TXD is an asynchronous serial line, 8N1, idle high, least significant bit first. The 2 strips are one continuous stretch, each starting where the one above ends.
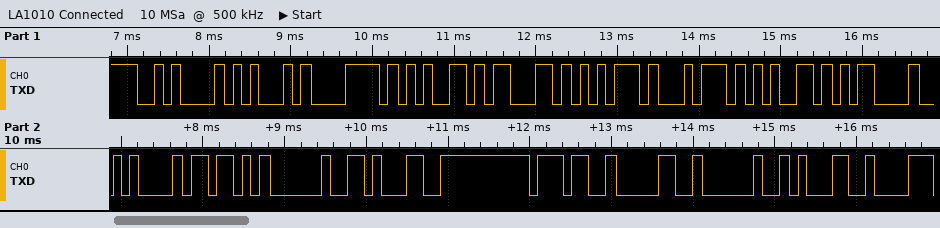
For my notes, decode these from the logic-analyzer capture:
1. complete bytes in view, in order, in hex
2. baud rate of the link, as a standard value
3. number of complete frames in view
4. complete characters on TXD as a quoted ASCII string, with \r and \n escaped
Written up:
0A 45 78 65 63 75 74 65 0D 0A 5B 20 31 37 30 20 31
9600 baud
17
"\nExecute\r\n[ 170 1"
